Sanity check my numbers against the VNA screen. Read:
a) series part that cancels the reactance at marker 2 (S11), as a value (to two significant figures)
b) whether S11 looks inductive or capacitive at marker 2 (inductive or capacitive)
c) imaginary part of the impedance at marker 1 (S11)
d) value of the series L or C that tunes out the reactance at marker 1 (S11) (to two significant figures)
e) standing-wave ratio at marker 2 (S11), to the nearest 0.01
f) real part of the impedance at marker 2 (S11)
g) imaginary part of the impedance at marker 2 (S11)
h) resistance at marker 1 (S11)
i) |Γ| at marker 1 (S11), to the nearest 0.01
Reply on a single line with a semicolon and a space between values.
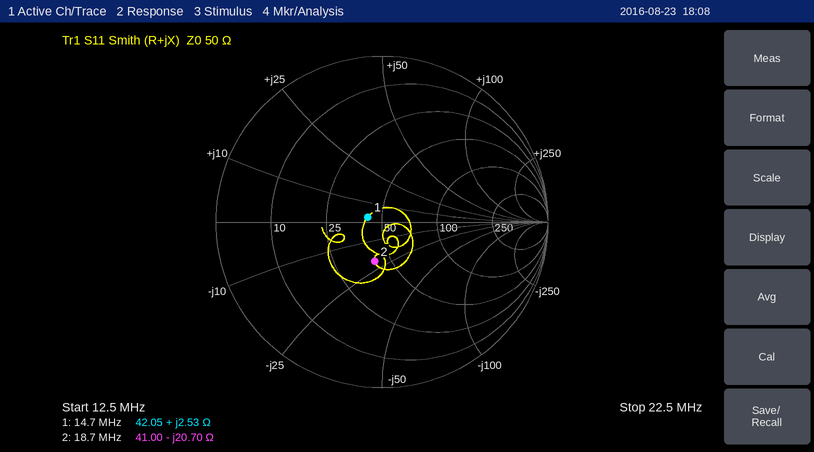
180 nH; capacitive; +2.53 Ω; 4.3 nF; 1.64; 41.00 Ω; -20.70 Ω; 42.05 Ω; 0.09
